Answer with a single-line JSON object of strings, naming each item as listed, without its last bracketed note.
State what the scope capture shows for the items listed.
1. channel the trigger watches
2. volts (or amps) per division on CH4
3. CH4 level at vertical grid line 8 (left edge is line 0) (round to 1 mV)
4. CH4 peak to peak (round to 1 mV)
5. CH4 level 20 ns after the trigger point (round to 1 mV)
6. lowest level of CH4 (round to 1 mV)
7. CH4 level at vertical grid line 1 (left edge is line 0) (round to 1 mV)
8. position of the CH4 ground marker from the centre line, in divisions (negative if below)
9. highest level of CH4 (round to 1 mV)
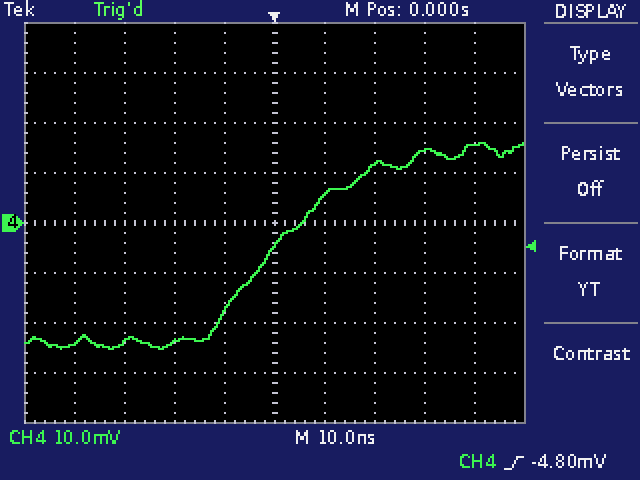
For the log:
{"channel the trigger watches": "CH4", "volts (or amps) per division on CH4": "10 mV", "CH4 level at vertical grid line 8 (left edge is line 0)": "15 mV", "CH4 peak to peak": "41 mV", "CH4 level 20 ns after the trigger point": "12 mV", "lowest level of CH4": "-25 mV", "CH4 level at vertical grid line 1 (left edge is line 0)": "-24 mV", "position of the CH4 ground marker from the centre line, in divisions": "0.0 div", "highest level of CH4": "16 mV"}
